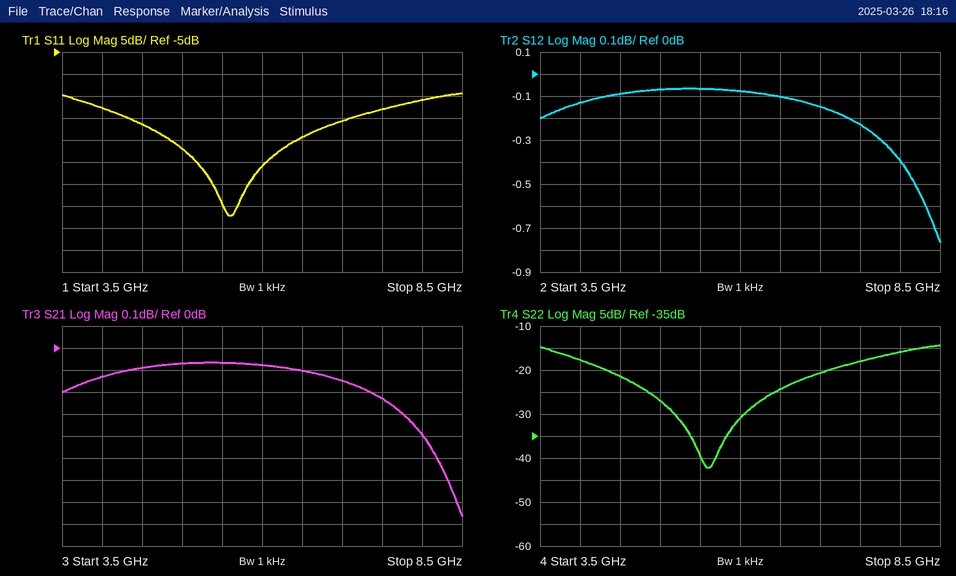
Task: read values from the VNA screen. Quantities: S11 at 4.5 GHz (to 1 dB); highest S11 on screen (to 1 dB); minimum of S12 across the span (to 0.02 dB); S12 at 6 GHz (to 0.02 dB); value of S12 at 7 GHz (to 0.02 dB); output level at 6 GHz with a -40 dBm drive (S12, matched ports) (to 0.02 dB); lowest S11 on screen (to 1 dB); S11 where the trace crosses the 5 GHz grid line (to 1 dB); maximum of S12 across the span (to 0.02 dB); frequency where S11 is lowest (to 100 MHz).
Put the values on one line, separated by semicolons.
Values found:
-21 dB; -14 dB; -0.76 dB; -0.08 dB; -0.14 dB; -40.08 dBm; -42 dB; -27 dB; -0.06 dB; 5.6 GHz
